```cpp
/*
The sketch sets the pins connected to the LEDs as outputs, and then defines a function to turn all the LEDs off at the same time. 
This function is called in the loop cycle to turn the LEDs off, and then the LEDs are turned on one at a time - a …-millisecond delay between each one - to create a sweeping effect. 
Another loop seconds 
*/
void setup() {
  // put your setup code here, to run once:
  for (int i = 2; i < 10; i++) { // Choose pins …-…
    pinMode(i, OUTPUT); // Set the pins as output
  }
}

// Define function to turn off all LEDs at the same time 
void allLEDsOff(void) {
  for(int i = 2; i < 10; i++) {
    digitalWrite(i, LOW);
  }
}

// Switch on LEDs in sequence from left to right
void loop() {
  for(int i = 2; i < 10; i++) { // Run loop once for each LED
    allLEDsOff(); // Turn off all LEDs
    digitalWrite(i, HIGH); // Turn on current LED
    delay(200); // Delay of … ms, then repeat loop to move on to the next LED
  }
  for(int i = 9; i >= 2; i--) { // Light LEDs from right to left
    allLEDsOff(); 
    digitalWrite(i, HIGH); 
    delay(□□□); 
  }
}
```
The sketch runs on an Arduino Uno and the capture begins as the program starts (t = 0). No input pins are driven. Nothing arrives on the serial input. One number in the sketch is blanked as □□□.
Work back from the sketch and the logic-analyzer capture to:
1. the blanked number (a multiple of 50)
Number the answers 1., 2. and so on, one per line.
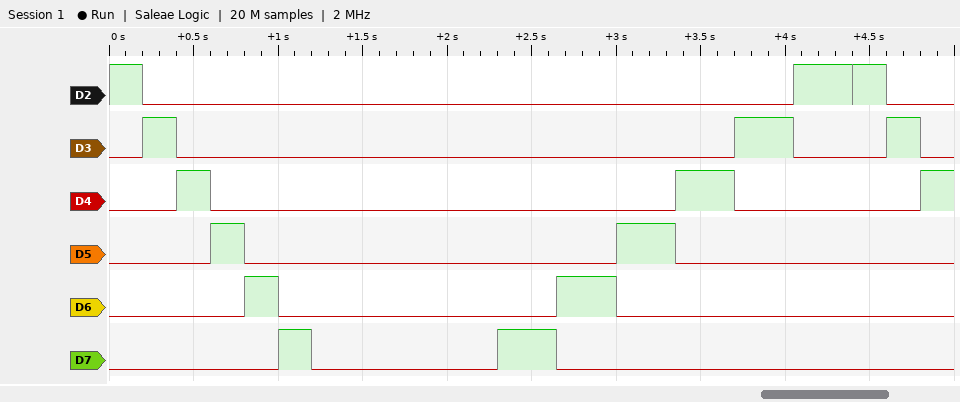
1. 350
